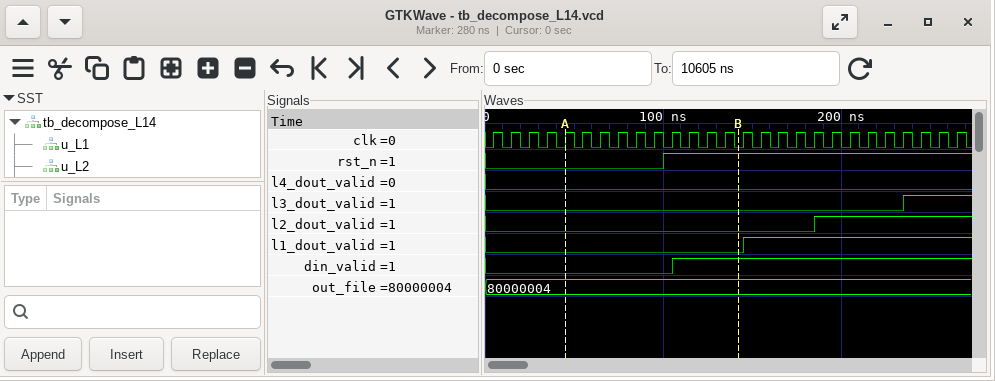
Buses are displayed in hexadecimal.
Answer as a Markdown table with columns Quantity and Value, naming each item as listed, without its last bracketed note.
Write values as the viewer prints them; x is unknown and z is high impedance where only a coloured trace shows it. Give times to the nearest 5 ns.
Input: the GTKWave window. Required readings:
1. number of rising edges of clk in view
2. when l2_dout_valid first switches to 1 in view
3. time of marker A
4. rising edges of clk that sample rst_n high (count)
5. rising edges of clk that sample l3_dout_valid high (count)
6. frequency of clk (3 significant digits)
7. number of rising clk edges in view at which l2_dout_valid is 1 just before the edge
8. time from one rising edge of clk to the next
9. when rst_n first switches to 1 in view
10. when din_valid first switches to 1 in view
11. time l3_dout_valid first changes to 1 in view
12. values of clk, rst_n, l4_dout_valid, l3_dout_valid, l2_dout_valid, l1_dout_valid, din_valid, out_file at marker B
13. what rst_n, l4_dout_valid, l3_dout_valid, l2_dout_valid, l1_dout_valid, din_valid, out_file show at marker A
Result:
| Quantity | Value |
|---|---|
| number of rising edges of clk in view | 27 |
| when l2_dout_valid first switches to 1 in view | 185 ns |
| time of marker A | 45 ns |
| rising edges of clk that sample rst_n high | 17 |
| rising edges of clk that sample l3_dout_valid high | 3 |
| frequency of clk | 100 MHz |
| number of rising clk edges in view at which l2_dout_valid is 1 just before the edge | 8 |
| time from one rising edge of clk to the next | 10 ns |
| when rst_n first switches to 1 in view | 100 ns |
| when din_valid first switches to 1 in view | 105 ns |
| time l3_dout_valid first changes to 1 in view | 235 ns |
| values of clk, rst_n, l4_dout_valid, l3_dout_valid, l2_dout_valid, l1_dout_valid, din_valid, out_file at marker B | clk=0, rst_n=1, l4_dout_valid=0, l3_dout_valid=0, l2_dout_valid=0, l1_dout_valid=0, din_valid=1, out_file=80000004 |
| what rst_n, l4_dout_valid, l3_dout_valid, l2_dout_valid, l1_dout_valid, din_valid, out_file show at marker A | rst_n=0, l4_dout_valid=0, l3_dout_valid=0, l2_dout_valid=0, l1_dout_valid=0, din_valid=0, out_file=80000004 |
